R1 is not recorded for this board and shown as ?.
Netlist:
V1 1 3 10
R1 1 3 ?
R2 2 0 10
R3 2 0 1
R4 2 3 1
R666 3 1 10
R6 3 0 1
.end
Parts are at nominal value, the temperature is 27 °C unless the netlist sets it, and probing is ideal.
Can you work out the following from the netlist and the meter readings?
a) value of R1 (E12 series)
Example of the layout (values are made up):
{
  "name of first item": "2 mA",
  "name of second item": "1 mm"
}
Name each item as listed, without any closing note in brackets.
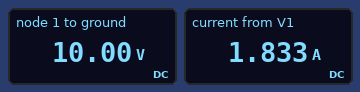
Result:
{
  "value of R1": "12 Ω"
}
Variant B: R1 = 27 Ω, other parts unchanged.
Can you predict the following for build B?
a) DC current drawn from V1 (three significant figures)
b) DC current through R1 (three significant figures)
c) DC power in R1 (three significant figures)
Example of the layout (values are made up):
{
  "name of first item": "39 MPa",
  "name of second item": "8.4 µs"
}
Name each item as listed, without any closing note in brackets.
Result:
{
  "DC current drawn from V1": "1.37 A",
  "DC current through R1": "370 mA",
  "DC power in R1": "3.70 W"
}
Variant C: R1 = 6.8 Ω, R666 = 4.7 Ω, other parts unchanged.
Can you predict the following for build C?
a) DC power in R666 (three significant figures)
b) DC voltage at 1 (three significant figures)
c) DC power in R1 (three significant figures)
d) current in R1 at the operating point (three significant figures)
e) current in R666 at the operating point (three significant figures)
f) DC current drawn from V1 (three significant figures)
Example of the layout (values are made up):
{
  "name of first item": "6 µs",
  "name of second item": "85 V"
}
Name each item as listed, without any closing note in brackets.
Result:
{
  "DC power in R666": "21.3 W",
  "DC voltage at 1": "10.0 V",
  "DC power in R1": "14.7 W",
  "current in R1 at the operating point": "1.47 A",
  "current in R666 at the operating point": "2.13 A",
  "DC current drawn from V1": "3.60 A"
}
